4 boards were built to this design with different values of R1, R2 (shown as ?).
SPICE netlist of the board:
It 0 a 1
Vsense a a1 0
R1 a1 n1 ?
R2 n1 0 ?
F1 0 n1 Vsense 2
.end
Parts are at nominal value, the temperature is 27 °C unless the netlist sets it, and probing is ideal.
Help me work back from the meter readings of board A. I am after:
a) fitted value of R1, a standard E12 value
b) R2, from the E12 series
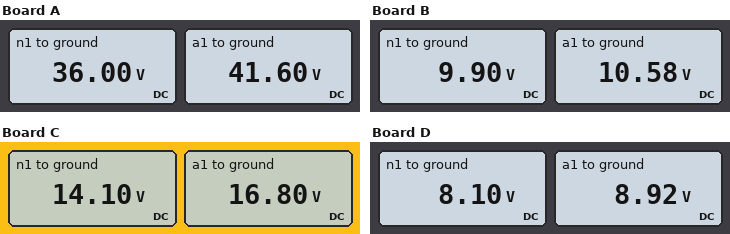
5.6 Ω
12 Ω
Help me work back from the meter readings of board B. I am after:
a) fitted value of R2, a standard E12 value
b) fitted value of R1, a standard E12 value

3.3 Ω
0.68 Ω
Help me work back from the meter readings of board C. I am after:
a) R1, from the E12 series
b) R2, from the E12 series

2.7 Ω
4.7 Ω
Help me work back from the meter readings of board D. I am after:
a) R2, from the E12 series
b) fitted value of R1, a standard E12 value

2.7 Ω
0.82 Ω
